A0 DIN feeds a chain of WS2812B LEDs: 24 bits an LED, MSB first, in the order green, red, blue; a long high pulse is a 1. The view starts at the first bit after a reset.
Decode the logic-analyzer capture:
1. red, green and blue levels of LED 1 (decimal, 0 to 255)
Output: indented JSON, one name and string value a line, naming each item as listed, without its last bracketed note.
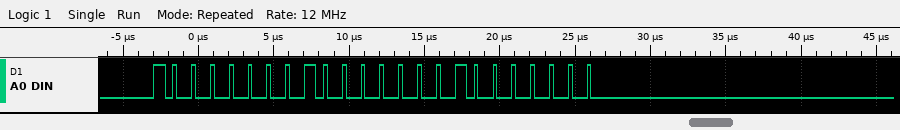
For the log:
{
  "red, green and blue levels of LED 1": "128, 128, 128"
}
